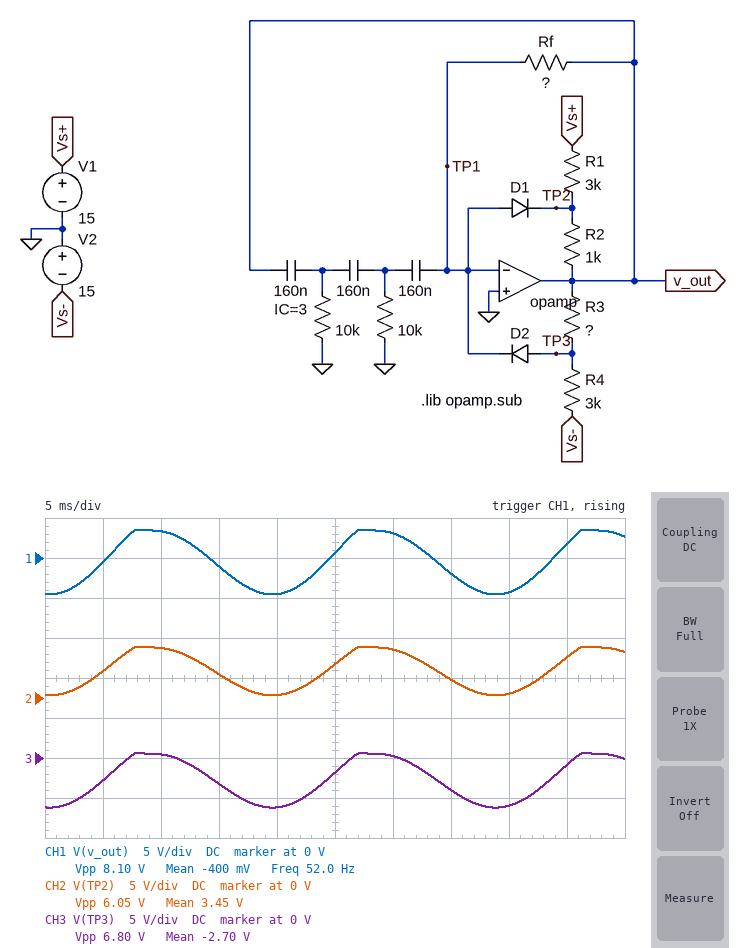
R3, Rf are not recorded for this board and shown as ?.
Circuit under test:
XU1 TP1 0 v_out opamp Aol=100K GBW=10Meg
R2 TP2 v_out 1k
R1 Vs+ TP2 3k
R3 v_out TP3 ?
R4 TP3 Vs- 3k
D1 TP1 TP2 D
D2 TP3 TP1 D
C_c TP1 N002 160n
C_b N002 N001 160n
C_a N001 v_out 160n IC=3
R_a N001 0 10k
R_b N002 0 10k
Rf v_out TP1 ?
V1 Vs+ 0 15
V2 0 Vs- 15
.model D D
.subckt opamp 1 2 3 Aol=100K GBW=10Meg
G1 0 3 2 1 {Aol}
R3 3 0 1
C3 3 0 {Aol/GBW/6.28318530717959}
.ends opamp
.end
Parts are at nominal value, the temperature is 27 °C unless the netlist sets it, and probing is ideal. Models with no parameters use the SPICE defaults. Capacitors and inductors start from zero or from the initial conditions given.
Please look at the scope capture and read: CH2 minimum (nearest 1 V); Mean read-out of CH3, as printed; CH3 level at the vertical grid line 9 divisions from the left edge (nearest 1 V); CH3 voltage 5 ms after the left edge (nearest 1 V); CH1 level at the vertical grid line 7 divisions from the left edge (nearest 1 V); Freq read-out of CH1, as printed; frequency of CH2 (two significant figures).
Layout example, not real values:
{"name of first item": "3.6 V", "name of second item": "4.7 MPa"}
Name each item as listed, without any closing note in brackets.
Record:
{"CH2 minimum": "0 V", "Mean read-out of CH3, as printed": "-2.70 V", "CH3 level at the vertical grid line 9 divisions from the left edge": "-1 V", "CH3 voltage 5 ms after the left edge": "-3 V", "CH1 level at the vertical grid line 7 divisions from the left edge": "-2 V", "Freq read-out of CH1, as printed": "52.0 Hz", "frequency of CH2": "52 Hz"}
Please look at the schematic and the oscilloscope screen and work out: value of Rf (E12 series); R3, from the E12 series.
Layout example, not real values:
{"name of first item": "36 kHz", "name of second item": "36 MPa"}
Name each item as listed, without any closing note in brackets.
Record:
{"value of Rf": "180 kΩ", "R3, from the E12 series": "560 Ω"}
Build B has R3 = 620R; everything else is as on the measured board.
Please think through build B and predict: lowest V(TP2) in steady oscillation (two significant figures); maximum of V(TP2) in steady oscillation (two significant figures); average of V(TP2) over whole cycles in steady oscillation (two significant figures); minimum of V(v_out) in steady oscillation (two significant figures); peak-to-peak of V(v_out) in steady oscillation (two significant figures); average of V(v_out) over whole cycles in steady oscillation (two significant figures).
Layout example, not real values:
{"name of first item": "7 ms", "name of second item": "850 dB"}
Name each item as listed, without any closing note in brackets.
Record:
{"lowest V(TP2) in steady oscillation": "20 mV", "maximum of V(TP2) in steady oscillation": "6.6 V", "average of V(TP2) over whole cycles in steady oscillation": "3.3 V", "minimum of V(v_out) in steady oscillation": "-5.0 V", "peak-to-peak of V(v_out) in steady oscillation": "8.8 V", "average of V(v_out) over whole cycles in steady oscillation": "-550 mV"}
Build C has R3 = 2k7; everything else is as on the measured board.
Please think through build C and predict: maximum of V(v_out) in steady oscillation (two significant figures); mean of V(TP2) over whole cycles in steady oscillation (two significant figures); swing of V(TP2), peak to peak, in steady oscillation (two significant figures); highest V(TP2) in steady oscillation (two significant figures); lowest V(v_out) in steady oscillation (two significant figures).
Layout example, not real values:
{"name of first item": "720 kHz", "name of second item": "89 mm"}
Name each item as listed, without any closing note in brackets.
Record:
{"maximum of V(v_out) in steady oscillation": "7.6 V", "mean of V(TP2) over whole cycles in steady oscillation": "4.4 V", "swing of V(TP2), peak to peak, in steady oscillation": "10 V", "highest V(TP2) in steady oscillation": "9.5 V", "lowest V(v_out) in steady oscillation": "-5.9 V"}
